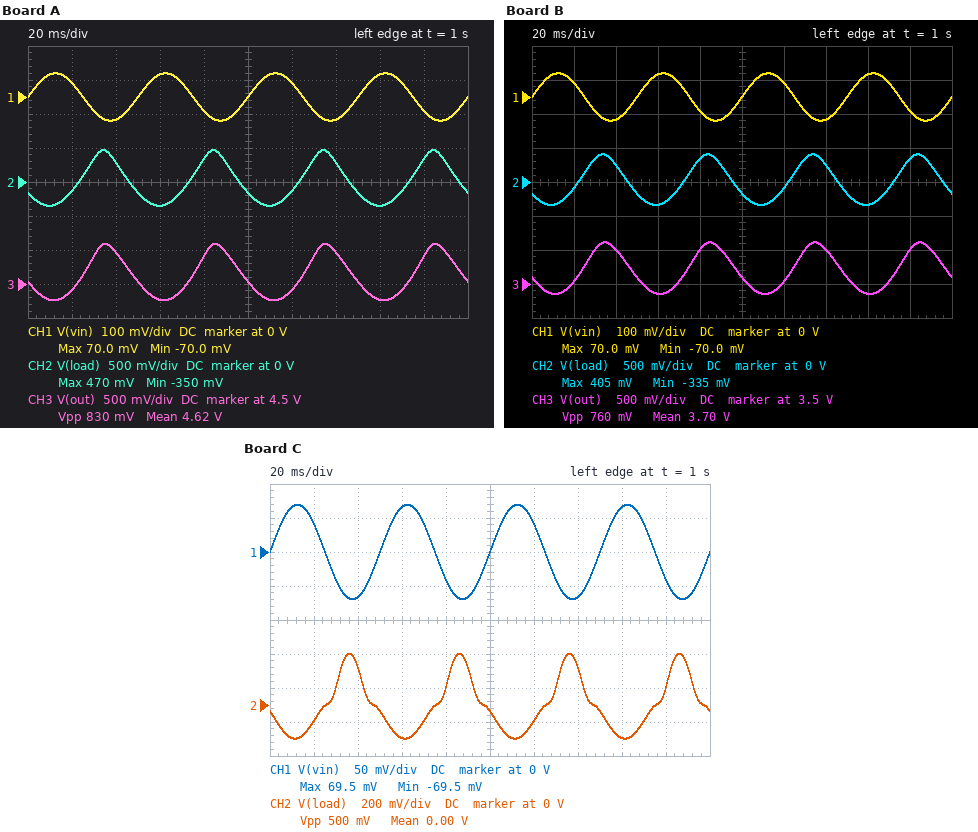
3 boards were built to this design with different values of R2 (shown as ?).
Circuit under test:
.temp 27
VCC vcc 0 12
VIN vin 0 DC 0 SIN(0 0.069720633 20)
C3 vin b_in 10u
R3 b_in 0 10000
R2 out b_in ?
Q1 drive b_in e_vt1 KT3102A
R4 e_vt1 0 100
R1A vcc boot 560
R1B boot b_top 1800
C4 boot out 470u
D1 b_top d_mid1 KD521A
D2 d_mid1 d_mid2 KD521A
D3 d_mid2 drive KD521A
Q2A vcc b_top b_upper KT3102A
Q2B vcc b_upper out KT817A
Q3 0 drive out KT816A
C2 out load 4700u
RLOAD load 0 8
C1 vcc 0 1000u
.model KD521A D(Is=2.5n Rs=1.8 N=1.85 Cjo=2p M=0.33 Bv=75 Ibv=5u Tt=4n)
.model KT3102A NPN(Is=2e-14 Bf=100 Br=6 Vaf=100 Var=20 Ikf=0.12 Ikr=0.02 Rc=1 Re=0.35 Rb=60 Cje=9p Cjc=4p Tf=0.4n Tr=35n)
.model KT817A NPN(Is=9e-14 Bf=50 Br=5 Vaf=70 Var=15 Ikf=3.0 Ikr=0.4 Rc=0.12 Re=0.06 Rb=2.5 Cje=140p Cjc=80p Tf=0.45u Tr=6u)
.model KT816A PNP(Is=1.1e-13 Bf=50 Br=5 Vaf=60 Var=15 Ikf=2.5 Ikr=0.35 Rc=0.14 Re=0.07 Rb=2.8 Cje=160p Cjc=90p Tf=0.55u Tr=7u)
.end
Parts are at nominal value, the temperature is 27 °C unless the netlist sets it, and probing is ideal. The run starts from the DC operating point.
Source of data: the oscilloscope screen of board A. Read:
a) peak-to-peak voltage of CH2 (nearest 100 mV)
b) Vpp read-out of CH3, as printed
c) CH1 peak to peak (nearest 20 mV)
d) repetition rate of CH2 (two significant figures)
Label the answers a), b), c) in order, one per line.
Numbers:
a) 800 mV
b) 830 mV
c) 140 mV
d) 20 Hz
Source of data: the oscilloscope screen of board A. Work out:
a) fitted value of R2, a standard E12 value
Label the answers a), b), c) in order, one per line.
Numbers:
a) 27 kΩ
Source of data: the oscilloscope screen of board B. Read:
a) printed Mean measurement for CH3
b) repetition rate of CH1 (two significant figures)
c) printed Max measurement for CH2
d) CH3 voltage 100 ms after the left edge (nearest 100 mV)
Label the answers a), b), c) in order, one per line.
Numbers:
a) 3.70 V
b) 20 Hz
c) 405 mV
d) 3.6 V
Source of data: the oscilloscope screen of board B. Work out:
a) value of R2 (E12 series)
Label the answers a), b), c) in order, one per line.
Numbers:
a) 18 kΩ
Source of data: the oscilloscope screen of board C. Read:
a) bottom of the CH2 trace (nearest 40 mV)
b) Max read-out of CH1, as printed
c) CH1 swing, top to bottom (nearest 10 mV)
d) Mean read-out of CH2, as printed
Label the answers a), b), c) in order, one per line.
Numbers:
a) -200 mV
b) 69.5 mV
c) 140 mV
d) 0.00 V
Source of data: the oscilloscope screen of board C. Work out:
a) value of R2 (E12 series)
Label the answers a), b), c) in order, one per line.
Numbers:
a) 150 kΩ
